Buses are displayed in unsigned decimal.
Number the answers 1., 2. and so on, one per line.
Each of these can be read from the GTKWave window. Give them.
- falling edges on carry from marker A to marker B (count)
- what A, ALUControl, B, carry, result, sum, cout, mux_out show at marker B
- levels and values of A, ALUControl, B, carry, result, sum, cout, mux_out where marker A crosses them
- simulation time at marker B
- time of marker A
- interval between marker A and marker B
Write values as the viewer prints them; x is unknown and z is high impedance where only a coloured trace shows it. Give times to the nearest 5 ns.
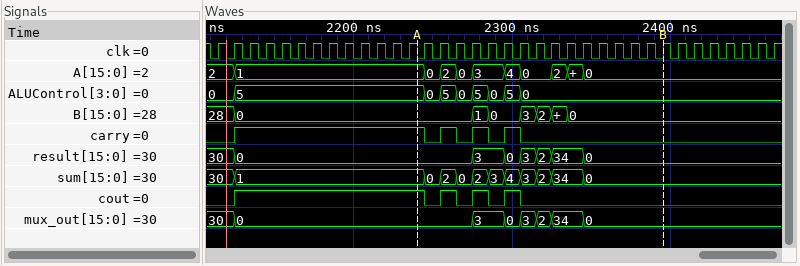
1. 4
2. A=0, ALUControl=0, B=0, carry=0, result=0, sum=0, cout=0, mux_out=0
3. A=1, ALUControl=5, B=0, carry=1, result=0, sum=1, cout=1, mux_out=0
4. 2395 ns
5. 2240 ns
6. 155 ns
